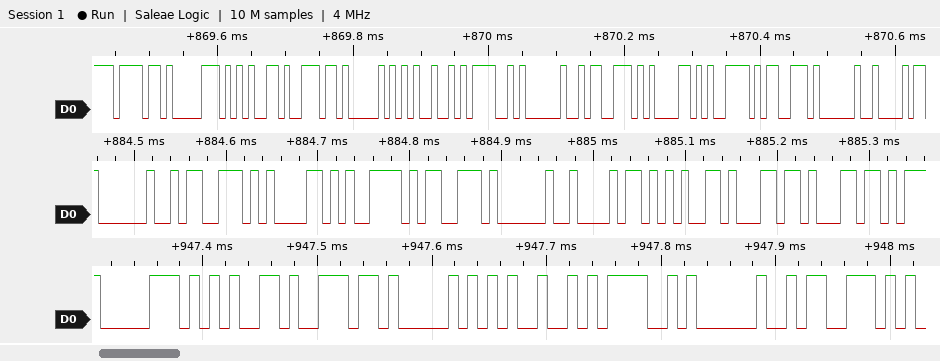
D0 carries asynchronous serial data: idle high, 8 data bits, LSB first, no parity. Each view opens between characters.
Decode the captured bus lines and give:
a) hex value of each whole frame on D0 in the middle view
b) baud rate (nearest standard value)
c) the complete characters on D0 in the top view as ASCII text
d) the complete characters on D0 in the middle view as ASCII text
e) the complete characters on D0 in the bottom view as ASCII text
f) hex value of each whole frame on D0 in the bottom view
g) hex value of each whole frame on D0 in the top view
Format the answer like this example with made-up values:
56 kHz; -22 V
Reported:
20, 73, 61, 79, 73, 20, 68, 65, 6C, 6C; 115200 baud; "openPIO says "; " says hell"; "penPIO s"; 70, 65, 6E, 50, 49, 4F, 20, 73; 6F, 70, 65, 6E, 50, 49, 4F, 20, 73, 61, 79, 73, 20
